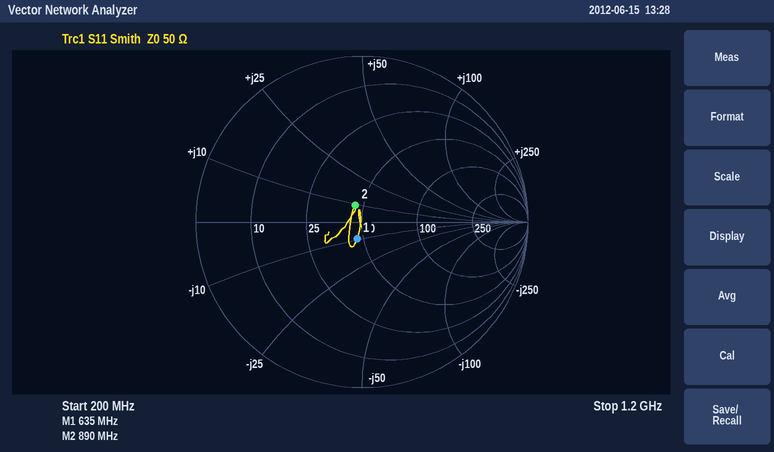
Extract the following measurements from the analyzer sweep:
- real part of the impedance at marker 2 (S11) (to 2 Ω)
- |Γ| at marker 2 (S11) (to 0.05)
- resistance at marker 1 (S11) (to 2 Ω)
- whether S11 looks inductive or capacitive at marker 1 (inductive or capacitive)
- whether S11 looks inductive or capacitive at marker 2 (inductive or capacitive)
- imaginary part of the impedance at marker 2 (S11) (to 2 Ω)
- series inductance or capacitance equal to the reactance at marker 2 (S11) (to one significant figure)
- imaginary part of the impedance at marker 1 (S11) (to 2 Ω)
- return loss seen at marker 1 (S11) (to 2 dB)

46 Ω
0.10
46 Ω
capacitive
inductive
+10 Ω
2 nH
-10 Ω
20 dB
